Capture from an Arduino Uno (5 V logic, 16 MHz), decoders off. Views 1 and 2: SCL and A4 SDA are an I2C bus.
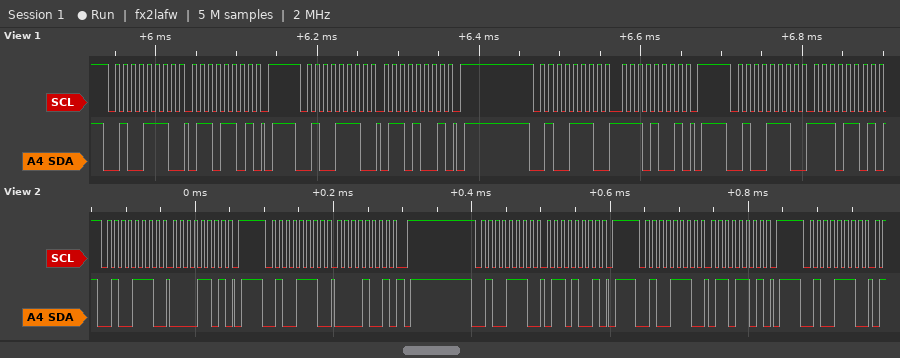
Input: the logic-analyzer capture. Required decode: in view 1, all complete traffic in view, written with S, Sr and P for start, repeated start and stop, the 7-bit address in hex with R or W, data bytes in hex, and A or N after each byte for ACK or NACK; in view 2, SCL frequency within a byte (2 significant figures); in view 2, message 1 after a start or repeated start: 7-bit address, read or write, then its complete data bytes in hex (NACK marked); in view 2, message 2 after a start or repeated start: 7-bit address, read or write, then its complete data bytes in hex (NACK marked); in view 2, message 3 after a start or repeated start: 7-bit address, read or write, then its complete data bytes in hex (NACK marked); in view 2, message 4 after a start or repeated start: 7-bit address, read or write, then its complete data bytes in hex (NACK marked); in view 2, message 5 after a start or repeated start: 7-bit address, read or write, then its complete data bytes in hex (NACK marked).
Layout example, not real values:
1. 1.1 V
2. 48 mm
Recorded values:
1. S 27W A 6D A P S 27W A 69 A P S 27W A E9 A P S 27W A ED A
2. 100 kHz
3. 0x27 write: 0D
4. 0x27 write: 09
5. 0x27 write: 69
6. 0x27 write: 6D
7. 0x27 write
